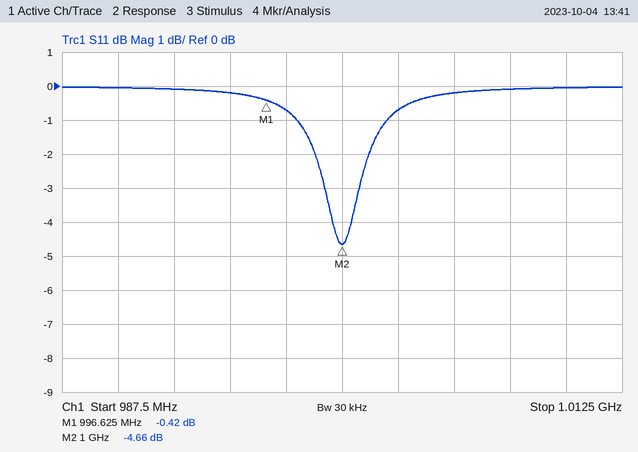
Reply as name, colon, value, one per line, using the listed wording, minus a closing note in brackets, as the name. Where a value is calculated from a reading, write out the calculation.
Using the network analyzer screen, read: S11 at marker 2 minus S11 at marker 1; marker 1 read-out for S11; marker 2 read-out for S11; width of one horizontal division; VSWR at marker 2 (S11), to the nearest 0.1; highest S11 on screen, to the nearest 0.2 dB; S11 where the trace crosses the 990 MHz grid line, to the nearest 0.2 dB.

S11 at marker 2 minus S11 at marker 1: -4.66 − (-0.42) = -4.24 dB
marker 1 read-out for S11: -0.42 dB
marker 2 read-out for S11: -4.66 dB
width of one horizontal division: 2.5 MHz
VSWR at marker 2 (S11), to the nearest 0.1: (1 + 0.5848)/(1 − 0.5848) ≈ 3.8
highest S11 on screen, to the nearest 0.2 dB: 0.0 dB
S11 where the trace crosses the 990 MHz grid line, to the nearest 0.2 dB: 0.0 dB
